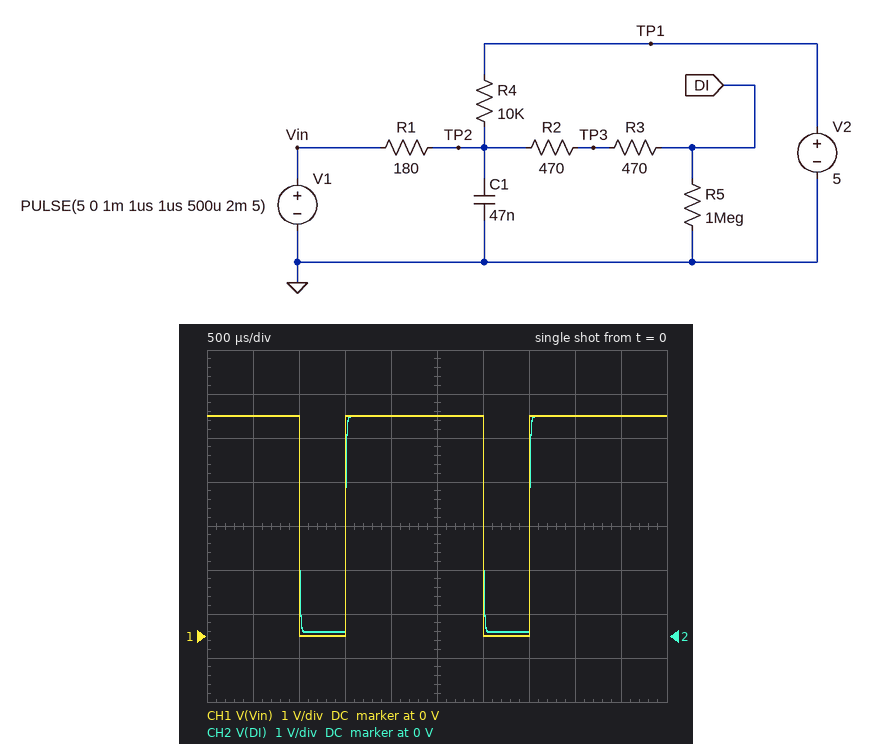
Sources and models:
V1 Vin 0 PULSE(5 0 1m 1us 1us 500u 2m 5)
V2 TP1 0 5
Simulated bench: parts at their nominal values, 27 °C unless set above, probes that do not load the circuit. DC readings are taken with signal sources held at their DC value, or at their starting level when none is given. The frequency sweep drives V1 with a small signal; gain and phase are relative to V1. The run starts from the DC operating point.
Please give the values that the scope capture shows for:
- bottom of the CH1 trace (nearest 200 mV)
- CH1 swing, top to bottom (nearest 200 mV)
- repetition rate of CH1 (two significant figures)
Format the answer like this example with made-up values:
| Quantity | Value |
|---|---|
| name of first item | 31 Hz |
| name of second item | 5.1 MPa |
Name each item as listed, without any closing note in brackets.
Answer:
| Quantity | Value |
|---|---|
| bottom of the CH1 trace | 0 V |
| CH1 swing, top to bottom | 5.0 V |
| repetition rate of CH1 | 500 Hz |
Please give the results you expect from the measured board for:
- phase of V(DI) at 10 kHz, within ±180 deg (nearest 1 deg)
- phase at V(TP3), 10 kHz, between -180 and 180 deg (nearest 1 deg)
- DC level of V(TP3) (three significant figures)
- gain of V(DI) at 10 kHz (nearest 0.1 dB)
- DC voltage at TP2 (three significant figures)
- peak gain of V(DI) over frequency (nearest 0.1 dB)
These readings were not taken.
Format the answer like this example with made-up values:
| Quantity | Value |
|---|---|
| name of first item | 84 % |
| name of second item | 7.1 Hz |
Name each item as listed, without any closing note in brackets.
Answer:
| Quantity | Value |
|---|---|
| phase of V(DI) at 10 kHz, within ±180 deg | -28 deg |
| phase at V(TP3), 10 kHz, between -180 and 180 deg | -28 deg |
| DC level of V(TP3) | 5.00 V |
| gain of V(DI) at 10 kHz | -1.2 dB |
| DC voltage at TP2 | 5.00 V |
| peak gain of V(DI) over frequency | -0.2 dB |
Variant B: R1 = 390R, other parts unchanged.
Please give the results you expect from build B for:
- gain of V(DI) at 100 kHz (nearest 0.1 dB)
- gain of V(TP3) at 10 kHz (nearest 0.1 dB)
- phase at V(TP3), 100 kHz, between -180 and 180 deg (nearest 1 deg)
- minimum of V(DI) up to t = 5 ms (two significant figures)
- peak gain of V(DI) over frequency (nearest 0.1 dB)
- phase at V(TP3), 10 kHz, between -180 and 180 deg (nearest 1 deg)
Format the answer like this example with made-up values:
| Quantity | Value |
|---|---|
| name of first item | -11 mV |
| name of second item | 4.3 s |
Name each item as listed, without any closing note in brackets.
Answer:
| Quantity | Value |
|---|---|
| gain of V(DI) at 100 kHz | -21.3 dB |
| gain of V(TP3) at 10 kHz | -3.8 dB |
| phase at V(TP3), 100 kHz, between -180 and 180 deg | -85 deg |
| minimum of V(DI) up to t = 5 ms | 190 mV |
| peak gain of V(DI) over frequency | -0.3 dB |
| phase at V(TP3), 10 kHz, between -180 and 180 deg | -48 deg |
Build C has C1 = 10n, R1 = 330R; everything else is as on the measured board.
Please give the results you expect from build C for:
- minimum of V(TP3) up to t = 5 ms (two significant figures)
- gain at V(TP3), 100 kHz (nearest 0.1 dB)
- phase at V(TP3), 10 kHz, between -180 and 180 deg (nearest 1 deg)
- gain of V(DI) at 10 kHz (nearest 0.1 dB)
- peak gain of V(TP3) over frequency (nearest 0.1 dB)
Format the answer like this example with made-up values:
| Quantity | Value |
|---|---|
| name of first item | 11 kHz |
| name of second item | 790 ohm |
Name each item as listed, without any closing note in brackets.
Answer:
| Quantity | Value |
|---|---|
| minimum of V(TP3) up to t = 5 ms | 160 mV |
| gain at V(TP3), 100 kHz | -7.3 dB |
| phase at V(TP3), 10 kHz, between -180 and 180 deg | -11 deg |
| gain of V(DI) at 10 kHz | -0.5 dB |
| peak gain of V(TP3) over frequency | -0.3 dB |
